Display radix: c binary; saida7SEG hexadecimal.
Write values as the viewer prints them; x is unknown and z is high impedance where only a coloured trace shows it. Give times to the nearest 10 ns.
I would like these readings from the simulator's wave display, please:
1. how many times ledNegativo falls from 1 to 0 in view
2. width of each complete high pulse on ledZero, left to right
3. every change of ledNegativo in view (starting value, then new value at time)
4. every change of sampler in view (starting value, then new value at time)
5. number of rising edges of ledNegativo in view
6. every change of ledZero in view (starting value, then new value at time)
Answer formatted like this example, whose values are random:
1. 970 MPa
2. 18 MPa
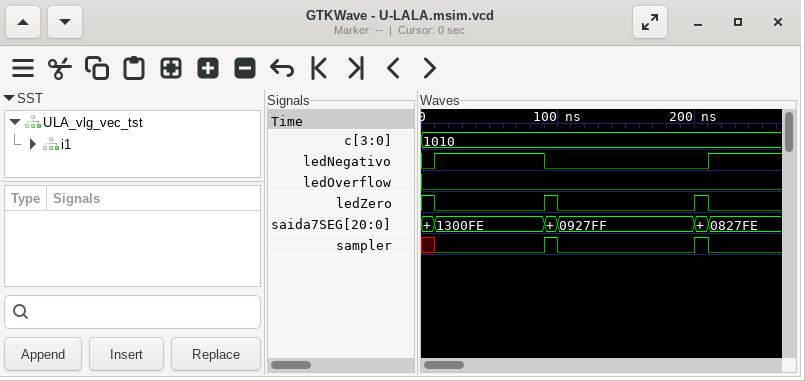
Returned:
1. 1
2. 10 ns, 10 ns
3. 0, 1 at 10 ns, 0 at 90 ns, 1 at 210 ns
4. x, 0 at 10 ns, 1 at 90 ns, 0 at 100 ns, 1 at 200 ns, 0 at 210 ns
5. 2
6. 1, 0 at 10 ns, 1 at 90 ns, 0 at 100 ns, 1 at 200 ns, 0 at 210 ns
